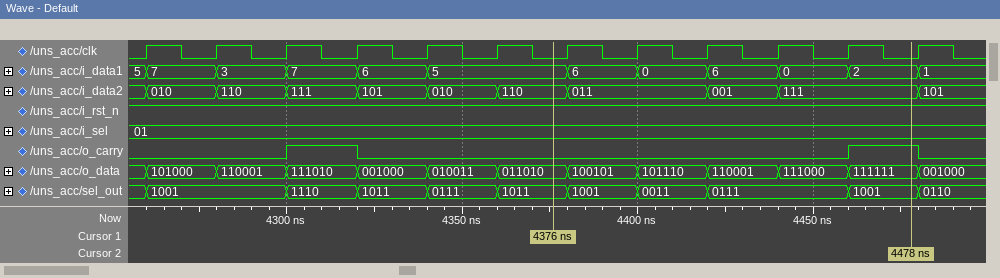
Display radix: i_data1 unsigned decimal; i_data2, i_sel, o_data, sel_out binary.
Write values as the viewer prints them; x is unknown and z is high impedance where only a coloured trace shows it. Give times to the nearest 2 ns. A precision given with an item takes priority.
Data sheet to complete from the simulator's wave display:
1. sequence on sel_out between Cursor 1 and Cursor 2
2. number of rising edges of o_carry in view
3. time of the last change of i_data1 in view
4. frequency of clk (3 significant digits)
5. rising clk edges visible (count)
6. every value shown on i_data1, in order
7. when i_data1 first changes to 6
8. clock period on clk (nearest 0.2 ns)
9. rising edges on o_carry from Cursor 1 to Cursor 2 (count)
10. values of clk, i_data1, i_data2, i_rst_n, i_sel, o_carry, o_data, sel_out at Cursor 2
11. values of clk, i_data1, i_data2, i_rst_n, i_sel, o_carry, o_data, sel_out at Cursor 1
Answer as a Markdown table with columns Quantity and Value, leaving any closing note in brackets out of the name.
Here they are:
| Quantity | Value |
|---|---|
| sequence on sel_out between Cursor 1 and Cursor 2 | 1011, 1001, 0011, 0111, 1001 |
| number of rising edges of o_carry in view | 2 |
| time of the last change of i_data1 in view | 4480 ns |
| frequency of clk | 50.0 MHz |
| rising clk edges visible | 12 |
| every value shown on i_data1, in order | 5, 7, 3, 7, 6, 5, 6, 0, 6, 0, 2, 1 |
| when i_data1 first changes to 6 | 4320 ns |
| clock period on clk | 20 ns |
| rising edges on o_carry from Cursor 1 to Cursor 2 | 1 |
| values of clk, i_data1, i_data2, i_rst_n, i_sel, o_carry, o_data, sel_out at Cursor 2 | clk=0, i_data1=2, i_data2=111, i_rst_n=1, i_sel=01, o_carry=1, o_data=111111, sel_out=1001 |
| values of clk, i_data1, i_data2, i_rst_n, i_sel, o_carry, o_data, sel_out at Cursor 1 | clk=0, i_data1=5, i_data2=110, i_rst_n=1, i_sel=01, o_carry=0, o_data=011010, sel_out=1011 |
